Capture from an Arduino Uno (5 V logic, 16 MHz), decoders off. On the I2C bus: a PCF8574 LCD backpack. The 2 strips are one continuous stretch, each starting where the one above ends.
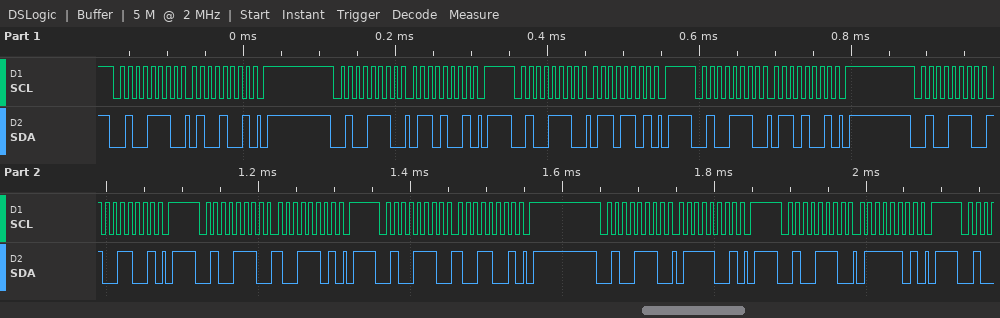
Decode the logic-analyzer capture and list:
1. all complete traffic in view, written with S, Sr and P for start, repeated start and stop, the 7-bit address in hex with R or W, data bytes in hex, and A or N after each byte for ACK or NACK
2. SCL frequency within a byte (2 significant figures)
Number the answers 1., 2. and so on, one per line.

1. S 27W A 49 A P S 27W A 69 A P S 27W A 6D A P S 27W A 69 A P S 27W A 99 A P S 27W A 9D A P S 27W A 99 A P S 27W A 79 A P S 27W A 7D A P
2. 100 kHz
